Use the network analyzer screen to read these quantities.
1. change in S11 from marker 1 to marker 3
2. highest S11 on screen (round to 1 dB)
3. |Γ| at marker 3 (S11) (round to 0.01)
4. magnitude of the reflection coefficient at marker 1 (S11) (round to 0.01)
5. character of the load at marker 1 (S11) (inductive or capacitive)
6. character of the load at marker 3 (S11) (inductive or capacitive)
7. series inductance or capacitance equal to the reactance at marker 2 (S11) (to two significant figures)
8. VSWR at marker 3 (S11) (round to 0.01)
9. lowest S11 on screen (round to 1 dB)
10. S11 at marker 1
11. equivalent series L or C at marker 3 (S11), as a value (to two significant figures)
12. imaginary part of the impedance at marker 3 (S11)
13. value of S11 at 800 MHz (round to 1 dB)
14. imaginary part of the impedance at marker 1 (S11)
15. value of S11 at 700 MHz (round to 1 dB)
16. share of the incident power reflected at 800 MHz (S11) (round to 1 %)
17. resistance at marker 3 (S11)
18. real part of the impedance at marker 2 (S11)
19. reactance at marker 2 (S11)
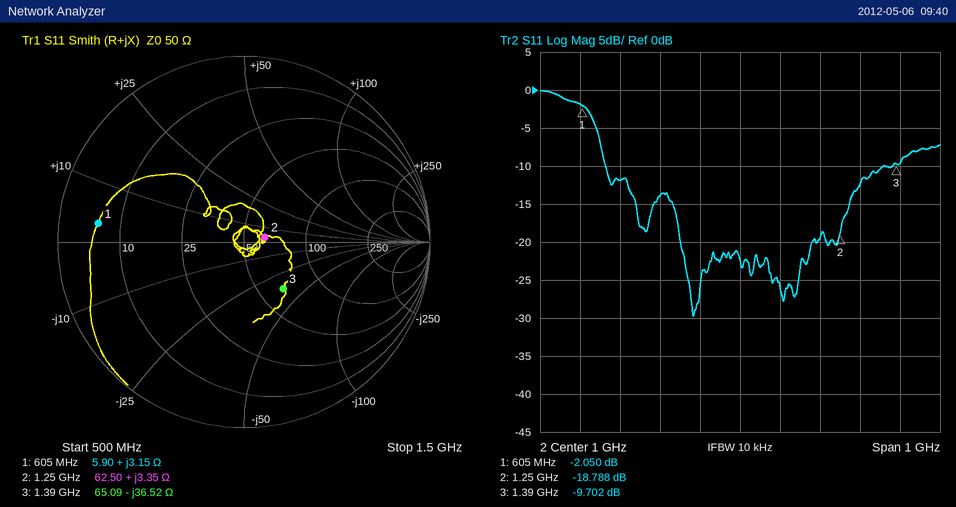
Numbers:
-7.652 dB
0 dB
0.33
0.79
inductive
capacitive
430 pH
1.97
-30 dB
-2.050 dB
3.1 pF
-36.52 Ω
-14 dB
+3.15 Ω
-12 dB
4 %
65.09 Ω
62.50 Ω
+3.35 Ω
